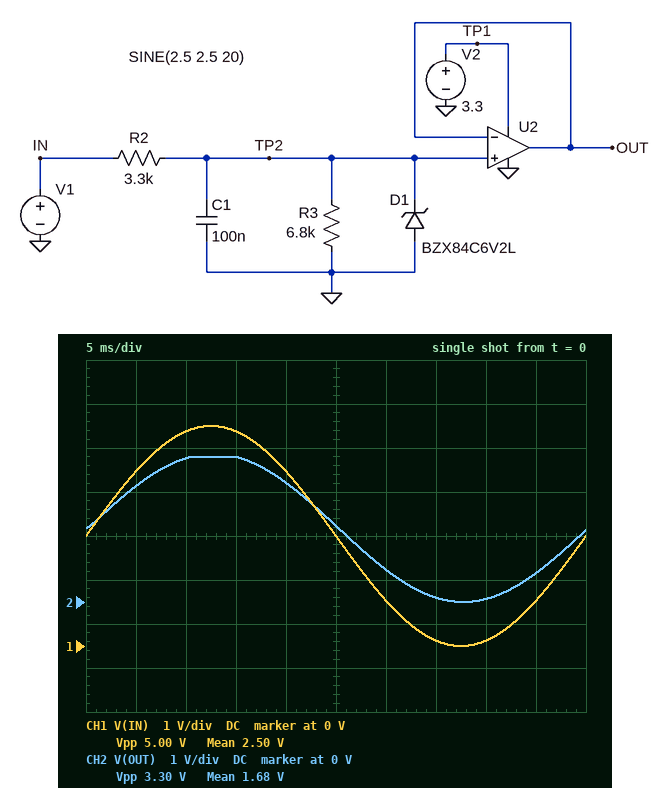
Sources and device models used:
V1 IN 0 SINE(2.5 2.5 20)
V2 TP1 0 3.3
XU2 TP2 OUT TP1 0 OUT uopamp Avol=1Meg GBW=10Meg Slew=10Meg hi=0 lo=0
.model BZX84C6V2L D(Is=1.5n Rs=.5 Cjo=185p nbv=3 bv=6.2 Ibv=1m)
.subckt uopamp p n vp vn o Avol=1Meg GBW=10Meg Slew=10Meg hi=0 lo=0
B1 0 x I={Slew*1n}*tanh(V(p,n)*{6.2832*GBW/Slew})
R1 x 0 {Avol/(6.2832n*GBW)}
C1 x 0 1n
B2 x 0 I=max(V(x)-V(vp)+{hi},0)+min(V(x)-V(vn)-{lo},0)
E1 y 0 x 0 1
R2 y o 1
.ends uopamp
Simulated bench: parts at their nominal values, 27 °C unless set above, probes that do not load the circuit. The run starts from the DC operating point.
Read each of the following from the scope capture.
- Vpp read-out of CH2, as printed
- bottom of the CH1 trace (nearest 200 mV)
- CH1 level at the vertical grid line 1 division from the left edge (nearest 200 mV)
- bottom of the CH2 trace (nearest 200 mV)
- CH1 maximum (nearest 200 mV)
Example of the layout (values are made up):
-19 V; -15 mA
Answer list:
3.30 V; 0 V; 4.0 V; 0 V; 5.0 V
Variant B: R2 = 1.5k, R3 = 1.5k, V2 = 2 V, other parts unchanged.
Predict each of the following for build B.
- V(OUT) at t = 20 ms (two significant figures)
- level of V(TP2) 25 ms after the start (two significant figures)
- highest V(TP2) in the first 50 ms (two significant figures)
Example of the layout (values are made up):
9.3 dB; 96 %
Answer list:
2.0 V; 1.3 V; 2.5 V
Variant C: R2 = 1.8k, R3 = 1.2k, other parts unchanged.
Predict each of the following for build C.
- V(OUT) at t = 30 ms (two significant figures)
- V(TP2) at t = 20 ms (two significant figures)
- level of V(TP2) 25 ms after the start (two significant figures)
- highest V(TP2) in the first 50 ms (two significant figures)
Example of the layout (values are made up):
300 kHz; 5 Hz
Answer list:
420 mV; 1.6 V; 1.0 V; 2.0 V
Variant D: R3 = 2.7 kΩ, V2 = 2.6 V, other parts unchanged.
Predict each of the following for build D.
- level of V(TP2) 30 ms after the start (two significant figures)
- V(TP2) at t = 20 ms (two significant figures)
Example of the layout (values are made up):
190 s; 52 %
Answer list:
480 mV; 1.8 V
